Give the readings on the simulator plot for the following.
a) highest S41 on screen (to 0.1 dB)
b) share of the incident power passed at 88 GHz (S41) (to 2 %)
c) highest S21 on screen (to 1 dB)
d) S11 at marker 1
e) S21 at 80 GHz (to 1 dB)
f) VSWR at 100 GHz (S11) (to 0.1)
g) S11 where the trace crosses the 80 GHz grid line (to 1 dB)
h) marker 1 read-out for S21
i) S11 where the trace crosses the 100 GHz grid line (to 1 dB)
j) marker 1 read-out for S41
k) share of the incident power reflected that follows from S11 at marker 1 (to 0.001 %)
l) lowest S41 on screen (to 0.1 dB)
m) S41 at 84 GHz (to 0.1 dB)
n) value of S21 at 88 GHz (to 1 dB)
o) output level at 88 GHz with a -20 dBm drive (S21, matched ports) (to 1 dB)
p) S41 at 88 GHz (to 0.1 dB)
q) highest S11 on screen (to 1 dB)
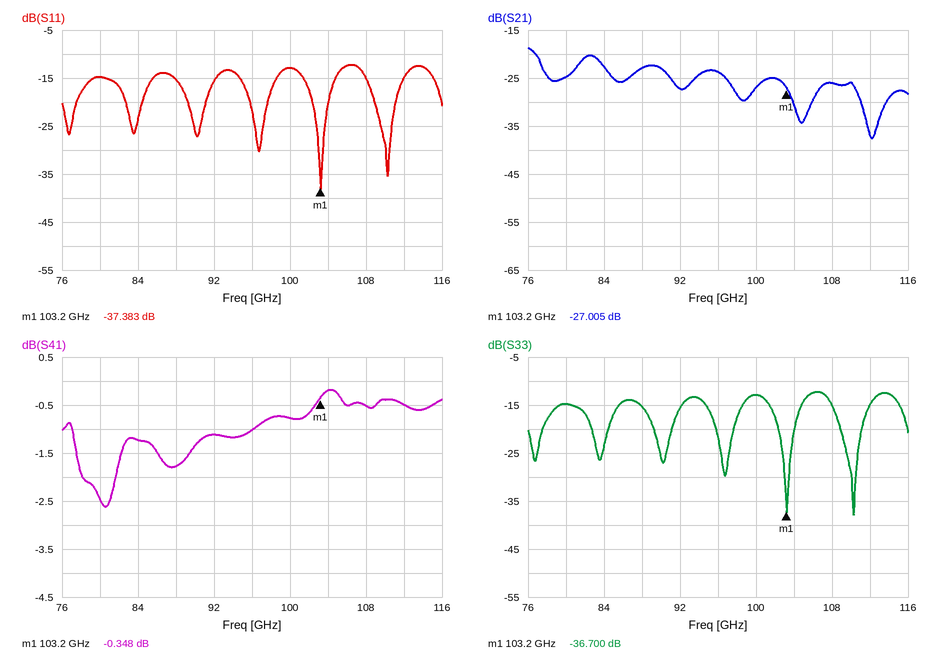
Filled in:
-0.2 dB
66 %
-19 dB
-37.383 dB
-25 dB
1.6
-15 dB
-27.005 dB
-13 dB
-0.348 dB
0.018 %
-2.6 dB
-1.2 dB
-23 dB
-43 dBm
-1.8 dB
-12 dB
